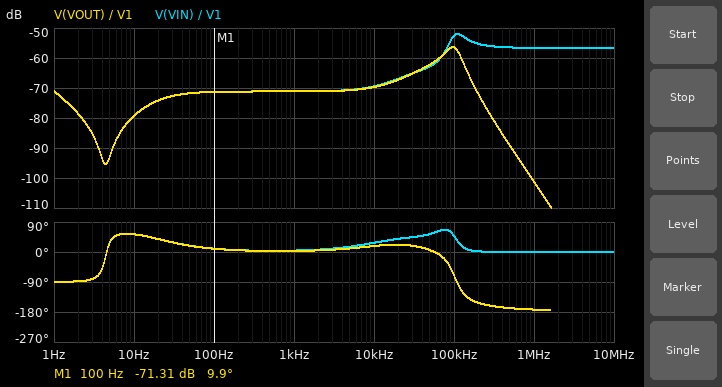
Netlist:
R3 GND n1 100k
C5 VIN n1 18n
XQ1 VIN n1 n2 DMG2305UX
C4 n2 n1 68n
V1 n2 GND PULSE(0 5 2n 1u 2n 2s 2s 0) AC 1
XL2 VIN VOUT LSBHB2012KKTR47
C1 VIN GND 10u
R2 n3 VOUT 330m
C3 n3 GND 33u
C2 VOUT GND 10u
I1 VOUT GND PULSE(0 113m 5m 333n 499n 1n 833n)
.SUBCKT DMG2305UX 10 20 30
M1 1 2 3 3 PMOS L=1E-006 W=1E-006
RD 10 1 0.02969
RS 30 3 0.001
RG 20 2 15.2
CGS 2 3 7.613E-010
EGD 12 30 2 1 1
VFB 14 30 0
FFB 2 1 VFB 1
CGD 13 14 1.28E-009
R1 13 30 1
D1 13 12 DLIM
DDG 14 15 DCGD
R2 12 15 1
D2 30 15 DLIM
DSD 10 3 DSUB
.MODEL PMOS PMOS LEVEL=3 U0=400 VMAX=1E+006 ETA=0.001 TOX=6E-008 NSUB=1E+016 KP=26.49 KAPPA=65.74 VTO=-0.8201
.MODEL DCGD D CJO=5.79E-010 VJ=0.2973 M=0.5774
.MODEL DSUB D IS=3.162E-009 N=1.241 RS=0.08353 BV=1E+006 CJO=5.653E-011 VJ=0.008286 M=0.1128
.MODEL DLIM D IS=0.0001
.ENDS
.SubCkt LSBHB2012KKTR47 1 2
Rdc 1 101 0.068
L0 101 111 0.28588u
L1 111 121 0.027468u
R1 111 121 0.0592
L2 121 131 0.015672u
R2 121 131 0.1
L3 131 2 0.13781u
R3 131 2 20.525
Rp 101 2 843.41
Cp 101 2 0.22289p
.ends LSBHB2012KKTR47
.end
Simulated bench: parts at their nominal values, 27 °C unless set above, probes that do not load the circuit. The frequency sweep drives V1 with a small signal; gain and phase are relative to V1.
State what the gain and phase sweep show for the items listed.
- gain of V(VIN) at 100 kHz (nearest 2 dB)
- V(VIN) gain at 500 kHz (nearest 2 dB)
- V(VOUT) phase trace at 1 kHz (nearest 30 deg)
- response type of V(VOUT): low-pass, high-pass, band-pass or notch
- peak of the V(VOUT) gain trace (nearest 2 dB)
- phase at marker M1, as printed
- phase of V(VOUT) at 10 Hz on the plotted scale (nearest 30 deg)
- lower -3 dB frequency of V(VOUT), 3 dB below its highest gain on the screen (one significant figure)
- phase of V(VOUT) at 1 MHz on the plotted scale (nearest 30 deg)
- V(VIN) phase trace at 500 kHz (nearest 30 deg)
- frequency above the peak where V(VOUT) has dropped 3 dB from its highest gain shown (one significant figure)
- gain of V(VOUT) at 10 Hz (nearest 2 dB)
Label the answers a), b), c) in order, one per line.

a) -52 dB
b) -56 dB
c) 0 deg
d) band-pass
e) -56 dB
f) 9.9 deg
g) 60 deg
h) 70 kHz
i) -180 deg
j) 0 deg
k) 100 kHz
l) -80 dB
